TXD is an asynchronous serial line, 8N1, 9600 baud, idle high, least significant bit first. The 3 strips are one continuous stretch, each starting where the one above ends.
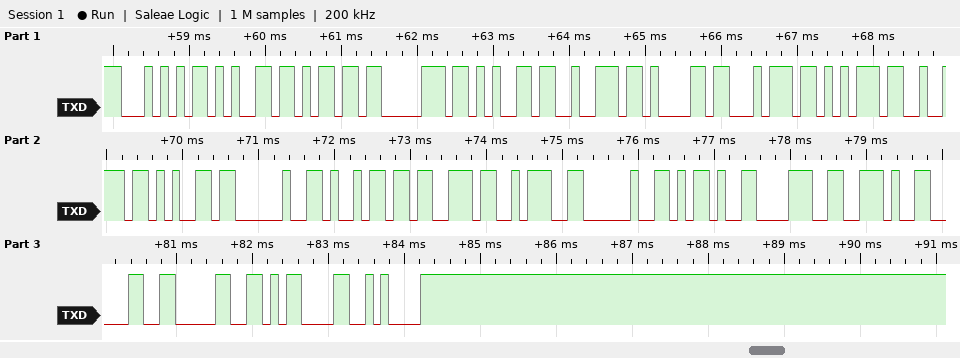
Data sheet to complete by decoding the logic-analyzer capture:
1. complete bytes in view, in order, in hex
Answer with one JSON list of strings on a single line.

["54 65 6D 70 65 72 61 74 75 72 65 20 69 73 3A 20 2D 38 2E 30 30 0D 0A"]
